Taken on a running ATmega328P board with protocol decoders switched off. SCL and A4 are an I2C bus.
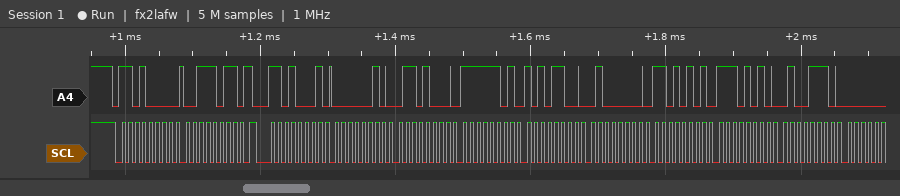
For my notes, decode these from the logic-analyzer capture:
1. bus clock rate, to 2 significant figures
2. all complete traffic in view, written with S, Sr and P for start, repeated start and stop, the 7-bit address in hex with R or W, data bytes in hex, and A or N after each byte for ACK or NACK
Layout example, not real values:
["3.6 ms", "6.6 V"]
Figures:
["100 kHz", "S 68W A 3B A Sr 68R A 02 A 68 A FD A AC A 40 A D5 A EA A 4E A"]
